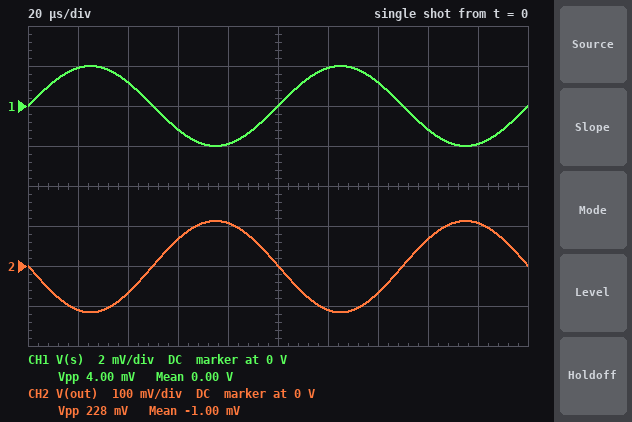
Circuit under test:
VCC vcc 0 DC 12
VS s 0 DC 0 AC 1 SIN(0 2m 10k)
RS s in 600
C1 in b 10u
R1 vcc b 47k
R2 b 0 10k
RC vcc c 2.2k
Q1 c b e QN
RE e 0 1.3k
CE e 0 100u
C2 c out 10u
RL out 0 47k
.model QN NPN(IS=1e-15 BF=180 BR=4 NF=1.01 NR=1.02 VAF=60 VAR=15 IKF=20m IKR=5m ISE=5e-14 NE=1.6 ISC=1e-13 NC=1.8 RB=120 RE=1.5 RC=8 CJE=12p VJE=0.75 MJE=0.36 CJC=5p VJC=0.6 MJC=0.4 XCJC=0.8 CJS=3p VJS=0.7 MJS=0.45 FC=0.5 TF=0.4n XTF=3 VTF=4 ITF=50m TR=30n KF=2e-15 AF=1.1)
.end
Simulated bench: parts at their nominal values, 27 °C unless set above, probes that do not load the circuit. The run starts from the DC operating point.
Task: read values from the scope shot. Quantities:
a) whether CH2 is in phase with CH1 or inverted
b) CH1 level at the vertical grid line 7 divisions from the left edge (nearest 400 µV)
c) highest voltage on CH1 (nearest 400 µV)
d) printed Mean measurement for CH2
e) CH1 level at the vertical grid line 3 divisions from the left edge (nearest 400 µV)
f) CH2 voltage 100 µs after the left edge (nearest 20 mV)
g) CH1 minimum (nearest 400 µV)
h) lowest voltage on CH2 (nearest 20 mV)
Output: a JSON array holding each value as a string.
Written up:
["inverted", "1.2 mV", "2.0 mV", "-1.00 mV", "-1.2 mV", "0 V", "-2.0 mV", "-120 mV"]
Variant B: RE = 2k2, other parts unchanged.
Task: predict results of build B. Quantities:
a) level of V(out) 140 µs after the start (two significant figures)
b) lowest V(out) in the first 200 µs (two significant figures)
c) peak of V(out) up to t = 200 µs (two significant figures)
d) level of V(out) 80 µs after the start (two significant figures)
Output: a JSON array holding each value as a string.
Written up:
["-46 mV", "-79 mV", "75 mV", "72 mV"]
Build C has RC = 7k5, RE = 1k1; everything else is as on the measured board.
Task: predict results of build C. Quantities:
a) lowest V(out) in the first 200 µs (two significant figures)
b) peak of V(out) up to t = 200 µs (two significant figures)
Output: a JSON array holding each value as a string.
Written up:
["-360 mV", "350 mV"]
